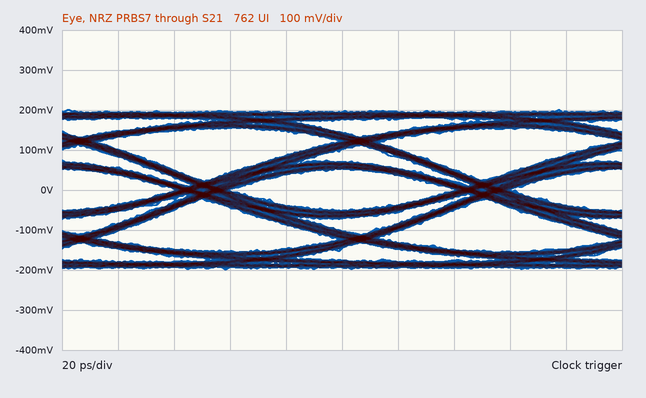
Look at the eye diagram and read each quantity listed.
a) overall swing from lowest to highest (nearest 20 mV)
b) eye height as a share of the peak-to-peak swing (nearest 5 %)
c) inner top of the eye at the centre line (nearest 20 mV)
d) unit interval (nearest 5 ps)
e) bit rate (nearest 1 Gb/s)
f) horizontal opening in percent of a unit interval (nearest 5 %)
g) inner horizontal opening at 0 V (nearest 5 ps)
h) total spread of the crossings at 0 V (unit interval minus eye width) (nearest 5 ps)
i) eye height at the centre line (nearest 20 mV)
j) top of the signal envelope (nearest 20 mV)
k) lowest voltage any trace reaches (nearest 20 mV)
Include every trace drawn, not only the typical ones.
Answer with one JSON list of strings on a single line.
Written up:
["400 mV", "25 %", "60 mV", "100 ps", "10 Gb/s", "80 %", "80 ps", "20 ps", "100 mV", "200 mV", "-200 mV"]
